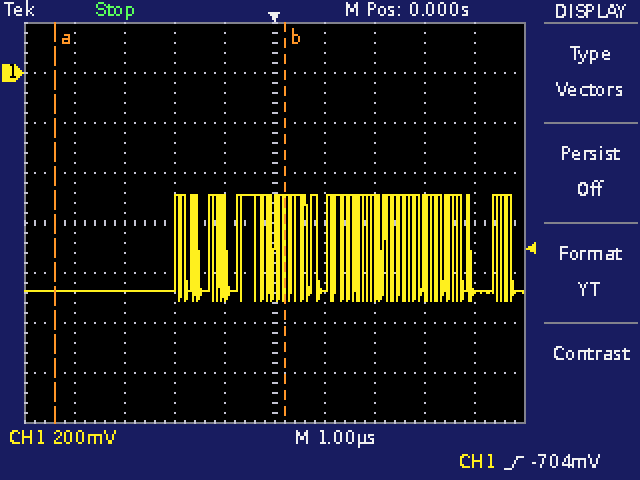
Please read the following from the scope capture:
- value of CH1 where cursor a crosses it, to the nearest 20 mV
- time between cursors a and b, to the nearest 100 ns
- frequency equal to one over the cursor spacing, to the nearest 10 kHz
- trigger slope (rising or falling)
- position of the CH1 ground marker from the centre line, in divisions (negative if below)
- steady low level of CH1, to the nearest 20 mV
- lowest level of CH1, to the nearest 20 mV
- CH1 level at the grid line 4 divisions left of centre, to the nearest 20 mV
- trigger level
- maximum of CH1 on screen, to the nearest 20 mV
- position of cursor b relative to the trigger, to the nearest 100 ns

-880 mV
4.6 µs
220 kHz
rising
+3.0 div
-880 mV
-920 mV
-880 mV
-704 mV
-480 mV
+200 ns
